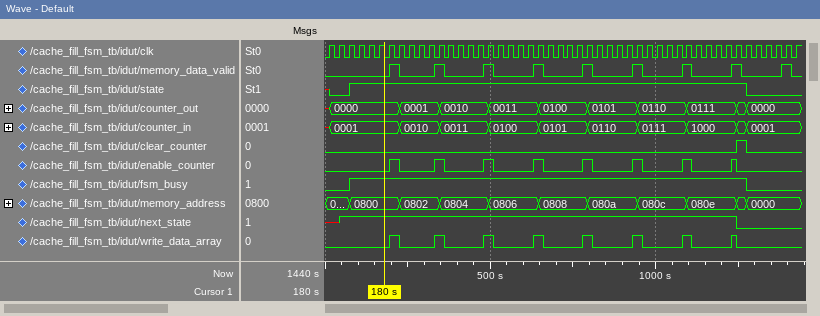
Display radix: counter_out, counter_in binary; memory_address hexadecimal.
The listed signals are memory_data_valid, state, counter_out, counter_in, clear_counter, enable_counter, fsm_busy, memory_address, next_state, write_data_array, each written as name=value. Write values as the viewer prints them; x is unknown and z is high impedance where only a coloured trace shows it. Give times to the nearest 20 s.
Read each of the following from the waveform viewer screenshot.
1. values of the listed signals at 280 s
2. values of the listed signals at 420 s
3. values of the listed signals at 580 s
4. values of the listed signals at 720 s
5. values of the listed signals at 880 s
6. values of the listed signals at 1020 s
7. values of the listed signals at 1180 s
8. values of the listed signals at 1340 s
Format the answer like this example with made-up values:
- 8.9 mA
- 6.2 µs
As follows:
- memory_data_valid=0, state=1, counter_out=0001, counter_in=0010, clear_counter=0, enable_counter=0, fsm_busy=1, memory_address=0802, next_state=1, write_data_array=0
- memory_data_valid=0, state=1, counter_out=0010, counter_in=0011, clear_counter=0, enable_counter=0, fsm_busy=1, memory_address=0804, next_state=1, write_data_array=0
- memory_data_valid=0, state=1, counter_out=0011, counter_in=0100, clear_counter=0, enable_counter=0, fsm_busy=1, memory_address=0806, next_state=1, write_data_array=0
- memory_data_valid=0, state=1, counter_out=0100, counter_in=0101, clear_counter=0, enable_counter=0, fsm_busy=1, memory_address=0808, next_state=1, write_data_array=0
- memory_data_valid=0, state=1, counter_out=0101, counter_in=0110, clear_counter=0, enable_counter=0, fsm_busy=1, memory_address=080a, next_state=1, write_data_array=0
- memory_data_valid=0, state=1, counter_out=0110, counter_in=0111, clear_counter=0, enable_counter=0, fsm_busy=1, memory_address=080c, next_state=1, write_data_array=0
- memory_data_valid=0, state=1, counter_out=0111, counter_in=1000, clear_counter=0, enable_counter=0, fsm_busy=1, memory_address=080e, next_state=1, write_data_array=0
- memory_data_valid=0, state=0, counter_out=0000, counter_in=0001, clear_counter=0, enable_counter=0, fsm_busy=0, memory_address=0000, next_state=0, write_data_array=0
